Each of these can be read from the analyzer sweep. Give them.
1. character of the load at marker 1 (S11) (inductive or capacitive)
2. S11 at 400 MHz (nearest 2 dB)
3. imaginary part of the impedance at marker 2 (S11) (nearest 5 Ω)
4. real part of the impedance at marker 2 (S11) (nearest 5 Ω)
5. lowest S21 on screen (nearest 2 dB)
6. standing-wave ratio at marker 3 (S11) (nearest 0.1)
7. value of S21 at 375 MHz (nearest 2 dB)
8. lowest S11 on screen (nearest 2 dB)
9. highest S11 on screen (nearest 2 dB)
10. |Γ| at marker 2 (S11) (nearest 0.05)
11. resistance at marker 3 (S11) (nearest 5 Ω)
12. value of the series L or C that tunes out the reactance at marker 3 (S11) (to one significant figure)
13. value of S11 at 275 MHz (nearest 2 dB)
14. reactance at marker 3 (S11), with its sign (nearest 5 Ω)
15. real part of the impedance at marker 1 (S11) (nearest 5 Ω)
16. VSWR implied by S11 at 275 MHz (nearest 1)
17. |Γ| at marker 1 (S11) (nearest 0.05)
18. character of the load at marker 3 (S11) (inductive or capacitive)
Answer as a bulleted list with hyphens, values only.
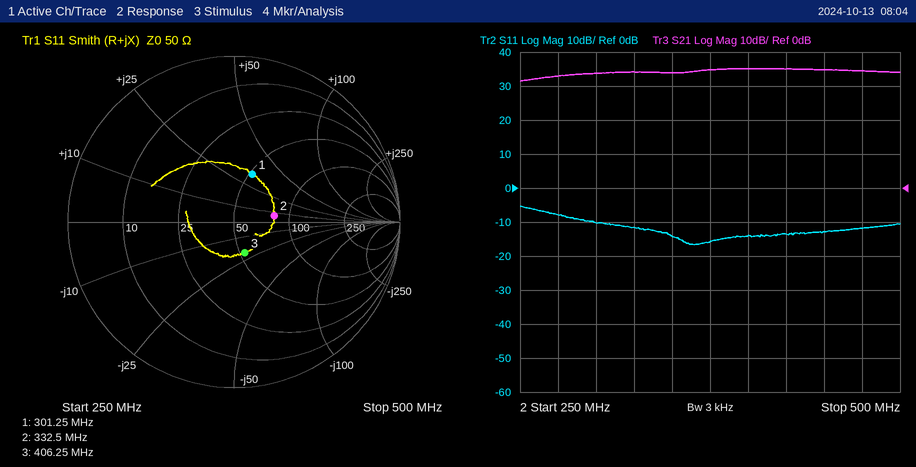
- inductive
- -14 dB
- +5 Ω
- 80 Ω
- 32 dB
- 1.5
- 34 dB
- -16 dB
- -6 dB
- 0.25
- 55 Ω
- 8 nH
- -8 dB
- -20 Ω
- 50 Ω
- 2
- 0.30
- capacitive
